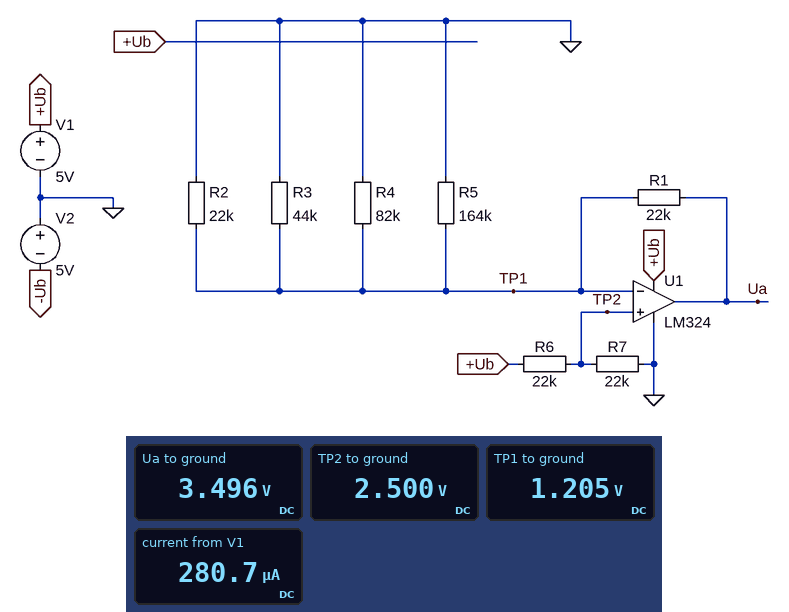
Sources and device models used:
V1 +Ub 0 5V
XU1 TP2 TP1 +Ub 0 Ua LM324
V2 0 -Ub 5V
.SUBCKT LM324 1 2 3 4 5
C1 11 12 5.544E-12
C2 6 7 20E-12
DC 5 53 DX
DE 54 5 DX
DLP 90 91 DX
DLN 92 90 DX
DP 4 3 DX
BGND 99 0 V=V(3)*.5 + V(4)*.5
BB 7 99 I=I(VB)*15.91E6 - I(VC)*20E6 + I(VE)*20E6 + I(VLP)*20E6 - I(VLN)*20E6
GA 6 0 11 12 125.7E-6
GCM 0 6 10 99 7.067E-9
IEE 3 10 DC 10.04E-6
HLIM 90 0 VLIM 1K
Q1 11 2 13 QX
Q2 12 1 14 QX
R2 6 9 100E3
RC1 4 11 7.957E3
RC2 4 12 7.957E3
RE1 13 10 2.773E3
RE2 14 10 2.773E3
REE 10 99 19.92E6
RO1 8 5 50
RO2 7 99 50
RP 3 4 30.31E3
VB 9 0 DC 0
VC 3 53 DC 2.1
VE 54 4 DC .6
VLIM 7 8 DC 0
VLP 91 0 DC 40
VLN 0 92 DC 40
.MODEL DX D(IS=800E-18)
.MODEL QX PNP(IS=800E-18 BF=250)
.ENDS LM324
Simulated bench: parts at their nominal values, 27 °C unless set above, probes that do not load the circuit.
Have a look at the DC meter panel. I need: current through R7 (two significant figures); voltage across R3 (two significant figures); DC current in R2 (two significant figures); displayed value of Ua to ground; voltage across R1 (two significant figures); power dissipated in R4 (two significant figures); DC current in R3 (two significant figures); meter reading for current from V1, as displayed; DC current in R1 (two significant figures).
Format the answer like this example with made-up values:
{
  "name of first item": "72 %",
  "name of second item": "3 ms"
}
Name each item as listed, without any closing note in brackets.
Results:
{
  "current through R7": "110 µA",
  "voltage across R3": "1.2 V",
  "DC current in R2": "55 µA",
  "displayed value of Ua to ground": "3.496 V",
  "voltage across R1": "2.3 V",
  "power dissipated in R4": "18 µW",
  "DC current in R3": "27 µA",
  "meter reading for current from V1, as displayed": "280.7 µA",
  "DC current in R1": "100 µA"
}
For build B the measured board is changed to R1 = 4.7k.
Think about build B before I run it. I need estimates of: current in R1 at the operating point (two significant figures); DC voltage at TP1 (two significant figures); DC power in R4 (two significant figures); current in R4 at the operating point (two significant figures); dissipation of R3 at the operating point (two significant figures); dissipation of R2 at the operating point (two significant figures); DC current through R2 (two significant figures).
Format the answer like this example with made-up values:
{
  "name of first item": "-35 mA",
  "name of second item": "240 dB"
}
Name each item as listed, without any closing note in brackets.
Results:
{
  "current in R1 at the operating point": "210 µA",
  "DC voltage at TP1": "2.5 V",
  "DC power in R4": "74 µW",
  "current in R4 at the operating point": "30 µA",
  "dissipation of R3 at the operating point": "140 µW",
  "dissipation of R2 at the operating point": "280 µW",
  "DC current through R2": "110 µA"
}
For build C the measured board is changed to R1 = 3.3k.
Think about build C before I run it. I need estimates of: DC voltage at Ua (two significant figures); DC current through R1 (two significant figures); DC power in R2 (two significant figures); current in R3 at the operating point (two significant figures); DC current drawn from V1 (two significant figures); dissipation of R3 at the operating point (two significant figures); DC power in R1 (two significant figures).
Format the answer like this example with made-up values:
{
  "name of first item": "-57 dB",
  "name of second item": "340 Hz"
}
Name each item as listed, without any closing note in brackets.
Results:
{
  "DC voltage at Ua": "3.2 V",
  "DC current through R1": "220 µA",
  "DC power in R2": "280 µW",
  "current in R3 at the operating point": "57 µA",
  "DC current drawn from V1": "290 µA",
  "dissipation of R3 at the operating point": "140 µW",
  "DC power in R1": "150 µW"
}
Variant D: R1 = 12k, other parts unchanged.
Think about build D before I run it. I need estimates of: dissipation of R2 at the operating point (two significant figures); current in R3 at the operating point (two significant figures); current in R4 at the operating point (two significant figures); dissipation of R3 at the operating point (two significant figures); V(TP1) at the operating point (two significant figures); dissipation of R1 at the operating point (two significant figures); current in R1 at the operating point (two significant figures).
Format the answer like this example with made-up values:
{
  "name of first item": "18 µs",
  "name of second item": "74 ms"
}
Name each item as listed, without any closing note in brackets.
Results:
{
  "dissipation of R2 at the operating point": "130 µW",
  "current in R3 at the operating point": "39 µA",
  "current in R4 at the operating point": "21 µA",
  "dissipation of R3 at the operating point": "67 µW",
  "V(TP1) at the operating point": "1.7 V",
  "dissipation of R1 at the operating point": "260 µW",
  "current in R1 at the operating point": "150 µA"
}
